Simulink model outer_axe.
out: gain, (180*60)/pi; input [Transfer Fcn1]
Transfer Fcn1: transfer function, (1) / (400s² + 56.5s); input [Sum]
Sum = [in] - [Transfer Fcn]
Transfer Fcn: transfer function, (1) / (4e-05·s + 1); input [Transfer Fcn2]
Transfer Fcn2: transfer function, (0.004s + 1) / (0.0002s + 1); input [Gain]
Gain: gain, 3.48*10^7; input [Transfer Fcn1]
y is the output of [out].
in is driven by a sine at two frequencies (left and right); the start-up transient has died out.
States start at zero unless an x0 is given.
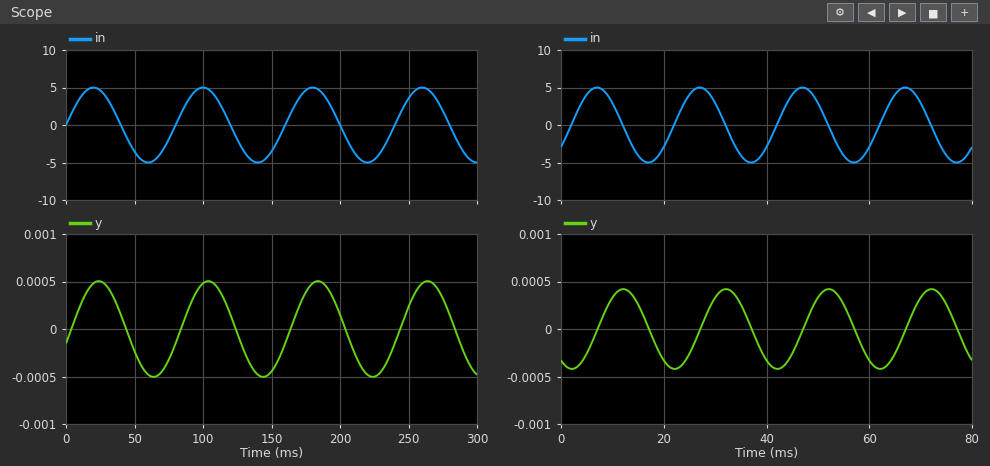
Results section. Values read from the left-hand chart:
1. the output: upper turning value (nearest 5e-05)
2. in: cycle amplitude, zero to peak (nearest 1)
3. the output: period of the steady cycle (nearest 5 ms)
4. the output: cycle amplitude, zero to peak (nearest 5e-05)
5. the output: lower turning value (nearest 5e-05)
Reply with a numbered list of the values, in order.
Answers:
1. 0.00050
2. 5
3. 80 ms
4. 0.00050
5. -0.00050
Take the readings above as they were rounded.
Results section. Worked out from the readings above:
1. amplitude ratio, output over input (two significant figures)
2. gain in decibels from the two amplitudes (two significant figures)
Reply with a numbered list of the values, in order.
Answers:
1. 0.00010
2. -80 dB
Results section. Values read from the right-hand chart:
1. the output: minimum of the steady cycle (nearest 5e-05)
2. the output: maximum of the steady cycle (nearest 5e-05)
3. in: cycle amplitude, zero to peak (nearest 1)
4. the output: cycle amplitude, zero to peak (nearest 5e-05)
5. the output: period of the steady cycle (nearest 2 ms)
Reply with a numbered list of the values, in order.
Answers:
1. -0.00040
2. 0.00040
3. 5
4. 0.00040
5. 20 ms
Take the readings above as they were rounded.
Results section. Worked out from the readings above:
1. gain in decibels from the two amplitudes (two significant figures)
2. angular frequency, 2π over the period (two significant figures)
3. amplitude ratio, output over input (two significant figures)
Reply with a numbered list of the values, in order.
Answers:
1. -82 dB
2. 0.31 rad/ms
3. 0.000080
